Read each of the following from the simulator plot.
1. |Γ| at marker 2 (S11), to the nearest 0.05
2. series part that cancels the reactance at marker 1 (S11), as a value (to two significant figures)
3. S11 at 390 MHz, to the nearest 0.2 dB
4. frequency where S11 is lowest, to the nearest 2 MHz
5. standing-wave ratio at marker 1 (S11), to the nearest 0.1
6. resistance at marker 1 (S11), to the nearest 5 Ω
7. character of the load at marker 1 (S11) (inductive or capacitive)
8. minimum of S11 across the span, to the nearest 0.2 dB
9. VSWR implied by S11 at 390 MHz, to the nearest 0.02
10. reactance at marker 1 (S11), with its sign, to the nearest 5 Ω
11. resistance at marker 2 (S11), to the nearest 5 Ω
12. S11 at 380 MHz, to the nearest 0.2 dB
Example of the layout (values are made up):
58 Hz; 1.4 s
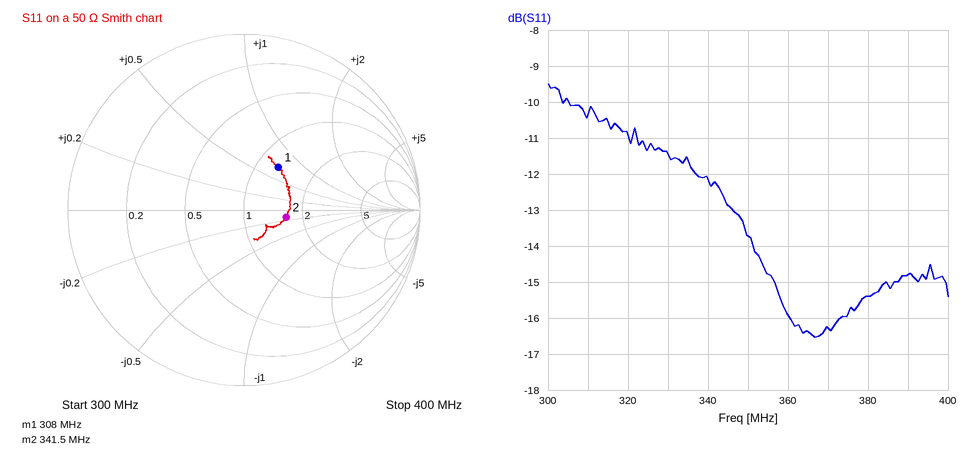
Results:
0.25; 15 pF; -14.8 dB; 366 MHz; 1.9; 65 Ω; inductive; -16.6 dB; 1.44; +35 Ω; 80 Ω; -15.4 dB
